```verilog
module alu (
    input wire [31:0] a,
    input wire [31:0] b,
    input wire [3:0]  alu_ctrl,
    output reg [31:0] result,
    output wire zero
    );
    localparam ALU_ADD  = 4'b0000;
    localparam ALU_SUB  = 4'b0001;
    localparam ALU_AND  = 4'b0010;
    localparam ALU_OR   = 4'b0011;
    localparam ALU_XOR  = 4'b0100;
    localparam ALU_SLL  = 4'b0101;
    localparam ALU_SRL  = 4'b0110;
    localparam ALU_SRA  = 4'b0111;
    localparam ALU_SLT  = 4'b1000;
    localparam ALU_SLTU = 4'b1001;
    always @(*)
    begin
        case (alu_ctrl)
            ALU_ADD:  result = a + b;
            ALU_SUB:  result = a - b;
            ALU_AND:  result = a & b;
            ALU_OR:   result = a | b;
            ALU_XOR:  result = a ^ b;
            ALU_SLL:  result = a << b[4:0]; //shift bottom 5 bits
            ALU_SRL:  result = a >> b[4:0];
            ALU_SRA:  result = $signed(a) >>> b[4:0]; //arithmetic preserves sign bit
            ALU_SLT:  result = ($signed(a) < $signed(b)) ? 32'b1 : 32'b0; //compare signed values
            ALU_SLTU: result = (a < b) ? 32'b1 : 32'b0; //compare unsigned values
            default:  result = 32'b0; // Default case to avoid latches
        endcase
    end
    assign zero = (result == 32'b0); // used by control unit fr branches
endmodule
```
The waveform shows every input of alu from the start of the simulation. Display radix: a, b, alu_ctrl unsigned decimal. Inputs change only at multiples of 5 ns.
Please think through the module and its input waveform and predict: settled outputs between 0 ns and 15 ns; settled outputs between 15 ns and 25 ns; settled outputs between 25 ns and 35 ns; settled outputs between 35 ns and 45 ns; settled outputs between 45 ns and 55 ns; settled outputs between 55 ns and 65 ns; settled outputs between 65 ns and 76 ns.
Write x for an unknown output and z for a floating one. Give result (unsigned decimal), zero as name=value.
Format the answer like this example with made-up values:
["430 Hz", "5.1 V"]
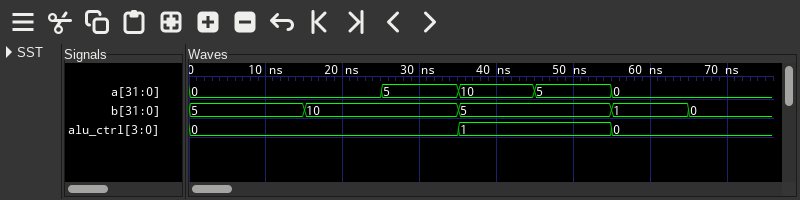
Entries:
["result=5, zero=0", "result=10, zero=0", "result=15, zero=0", "result=5, zero=0", "result=0, zero=1", "result=1, zero=0", "result=0, zero=1"]
